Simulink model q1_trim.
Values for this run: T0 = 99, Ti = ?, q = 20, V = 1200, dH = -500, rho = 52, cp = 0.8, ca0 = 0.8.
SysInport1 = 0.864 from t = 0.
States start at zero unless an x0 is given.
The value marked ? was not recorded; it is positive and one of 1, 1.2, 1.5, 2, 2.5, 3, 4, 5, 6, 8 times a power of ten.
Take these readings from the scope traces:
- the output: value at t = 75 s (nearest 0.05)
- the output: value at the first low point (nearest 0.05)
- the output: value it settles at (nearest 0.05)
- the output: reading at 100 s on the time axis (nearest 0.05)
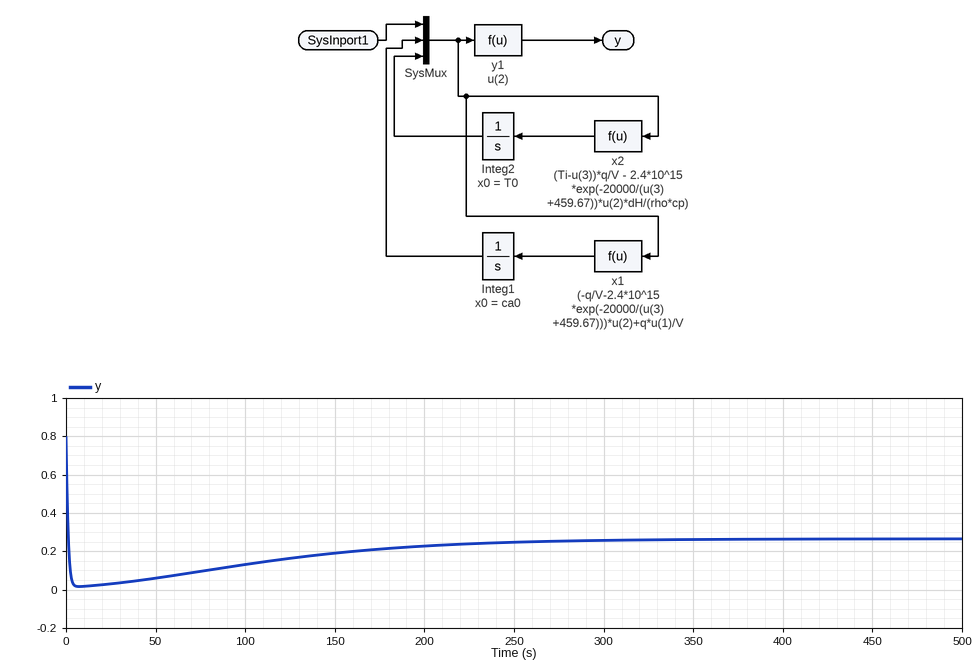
0.10
0.00
0.25
0.15
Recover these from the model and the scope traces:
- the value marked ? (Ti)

50
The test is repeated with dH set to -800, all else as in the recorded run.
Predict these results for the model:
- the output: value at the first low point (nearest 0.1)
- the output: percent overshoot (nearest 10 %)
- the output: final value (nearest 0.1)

0.0
30 %
0.2
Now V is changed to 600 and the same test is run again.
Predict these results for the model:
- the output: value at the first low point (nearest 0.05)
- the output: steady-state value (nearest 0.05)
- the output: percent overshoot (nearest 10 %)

0.05
0.45
110 %
